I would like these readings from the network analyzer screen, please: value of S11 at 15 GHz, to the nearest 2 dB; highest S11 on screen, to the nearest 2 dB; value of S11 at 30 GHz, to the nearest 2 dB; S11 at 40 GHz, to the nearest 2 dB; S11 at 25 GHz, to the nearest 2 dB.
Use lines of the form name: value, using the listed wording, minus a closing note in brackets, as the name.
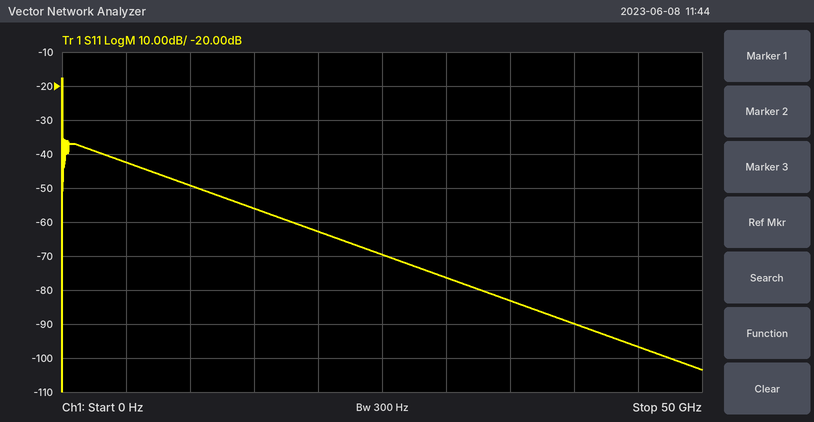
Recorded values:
value of S11 at 15 GHz, to the nearest 2 dB: -56 dB
highest S11 on screen, to the nearest 2 dB: -18 dB
value of S11 at 30 GHz, to the nearest 2 dB: -76 dB
S11 at 40 GHz, to the nearest 2 dB: -90 dB
S11 at 25 GHz, to the nearest 2 dB: -70 dB
